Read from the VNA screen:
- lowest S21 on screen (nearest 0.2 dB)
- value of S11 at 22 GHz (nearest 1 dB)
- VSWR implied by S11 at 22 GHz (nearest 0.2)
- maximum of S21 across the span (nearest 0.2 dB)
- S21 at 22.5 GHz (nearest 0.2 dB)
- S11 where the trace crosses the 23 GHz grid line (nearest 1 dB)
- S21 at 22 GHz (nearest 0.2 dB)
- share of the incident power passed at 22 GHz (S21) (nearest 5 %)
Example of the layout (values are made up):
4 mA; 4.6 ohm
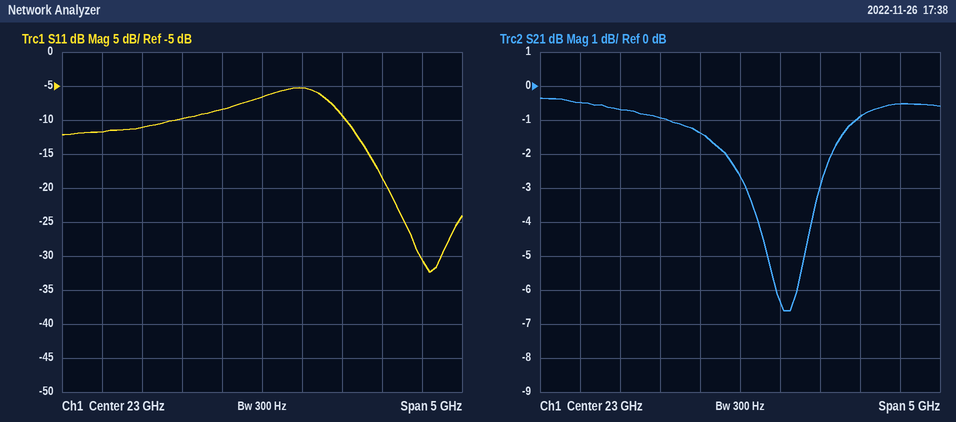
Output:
-6.6 dB; -10 dB; 2.0; -0.4 dB; -1.4 dB; -7 dB; -1.0 dB; 80 %
